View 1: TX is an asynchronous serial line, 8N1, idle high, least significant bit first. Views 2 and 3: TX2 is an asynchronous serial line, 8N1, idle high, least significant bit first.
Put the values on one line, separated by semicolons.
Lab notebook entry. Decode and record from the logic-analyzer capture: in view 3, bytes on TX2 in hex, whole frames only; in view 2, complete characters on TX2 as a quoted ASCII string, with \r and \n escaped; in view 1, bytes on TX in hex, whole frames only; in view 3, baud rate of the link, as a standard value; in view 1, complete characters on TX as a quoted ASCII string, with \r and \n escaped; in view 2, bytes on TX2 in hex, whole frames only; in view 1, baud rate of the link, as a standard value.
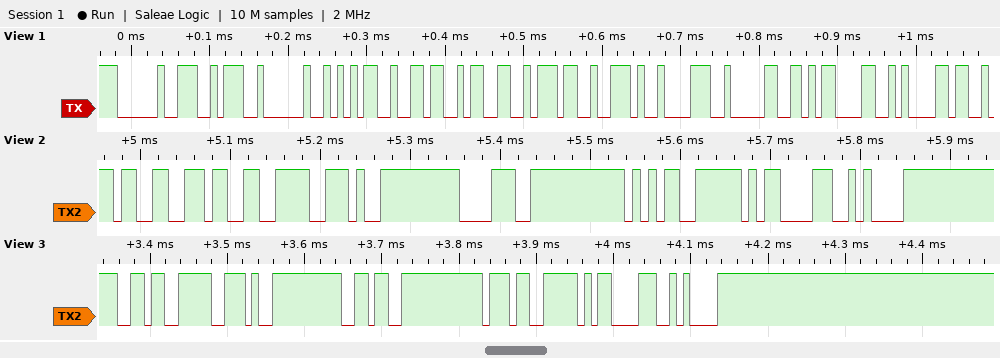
36 2E 36 37 0D 0A; "33.85\r\n"; 0x20 0x3A 0x20 0x35 0x36 0x33 0x37 0x2E 0x38 0x30 0x0D 0x0A; 115200 baud; " : 5637.80\r\n"; 33 33 2E 38 35 0D 0A; 115200 baud
